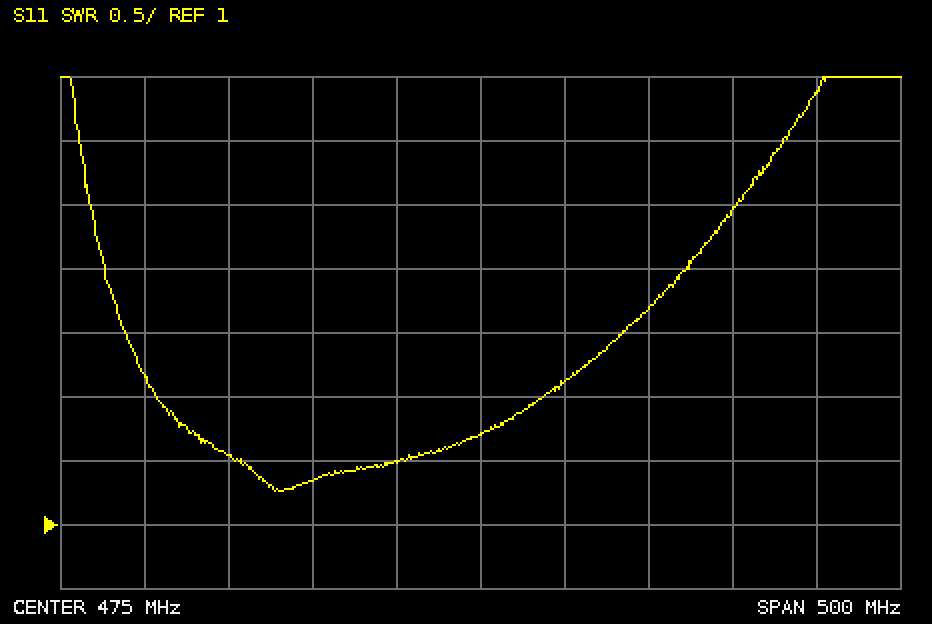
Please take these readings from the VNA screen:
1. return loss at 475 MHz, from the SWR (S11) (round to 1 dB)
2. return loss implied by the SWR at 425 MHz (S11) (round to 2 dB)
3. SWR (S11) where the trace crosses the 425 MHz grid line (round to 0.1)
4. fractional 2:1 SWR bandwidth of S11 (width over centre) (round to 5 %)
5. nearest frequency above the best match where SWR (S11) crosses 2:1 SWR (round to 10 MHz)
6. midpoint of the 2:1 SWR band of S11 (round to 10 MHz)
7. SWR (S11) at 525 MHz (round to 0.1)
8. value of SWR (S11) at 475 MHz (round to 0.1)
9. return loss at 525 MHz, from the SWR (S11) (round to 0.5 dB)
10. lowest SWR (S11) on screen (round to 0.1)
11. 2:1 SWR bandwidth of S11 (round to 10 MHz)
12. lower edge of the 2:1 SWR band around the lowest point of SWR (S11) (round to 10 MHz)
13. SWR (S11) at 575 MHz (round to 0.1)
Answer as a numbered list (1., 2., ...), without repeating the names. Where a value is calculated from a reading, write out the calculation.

1. −20 log10((1.7 − 1)/(1.7 + 1)) ≈ 12 dB
2. −20 log10((1.5 − 1)/(1.5 + 1)) ≈ 14 dB
3. 1.5
4. 230 MHz / 395 MHz ≈ 58.2 %, so 60 % to the nearest 5 %
5. 510 MHz
6. 400 MHz
7. 2.1
8. 1.7
9. −20 log10((2.1 − 1)/(2.1 + 1)) ≈ 9.0 dB
10. 1.3
11. 510 MHz − 280 MHz = 230 MHz
12. 280 MHz
13. 2.7
